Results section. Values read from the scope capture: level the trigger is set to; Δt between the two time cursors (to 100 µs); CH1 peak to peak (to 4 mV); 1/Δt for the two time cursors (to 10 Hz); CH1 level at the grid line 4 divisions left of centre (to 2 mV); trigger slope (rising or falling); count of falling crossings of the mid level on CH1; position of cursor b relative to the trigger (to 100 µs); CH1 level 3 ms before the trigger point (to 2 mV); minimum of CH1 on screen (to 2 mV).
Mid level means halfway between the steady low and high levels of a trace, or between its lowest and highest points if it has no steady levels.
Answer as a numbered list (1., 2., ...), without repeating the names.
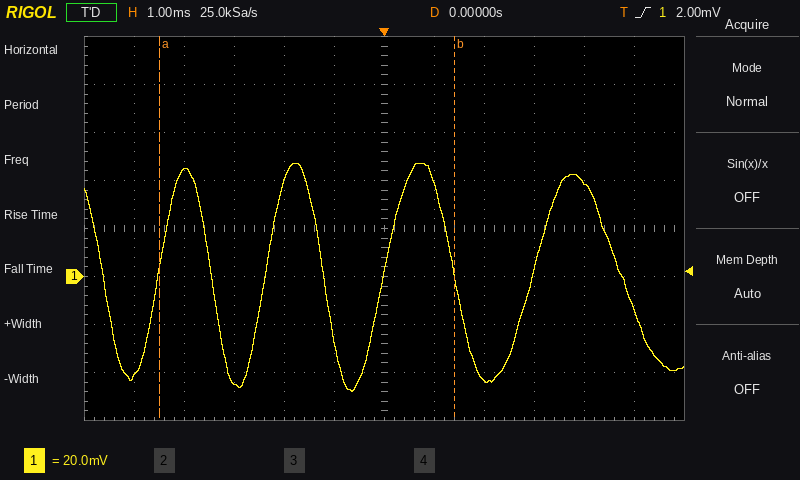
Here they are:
1. 2.00 mV
2. 5.9 ms
3. 96 mV
4. 170 Hz
5. 44 mV
6. rising
7. 5
8. +1.4 ms
9. -44 mV
10. -48 mV
